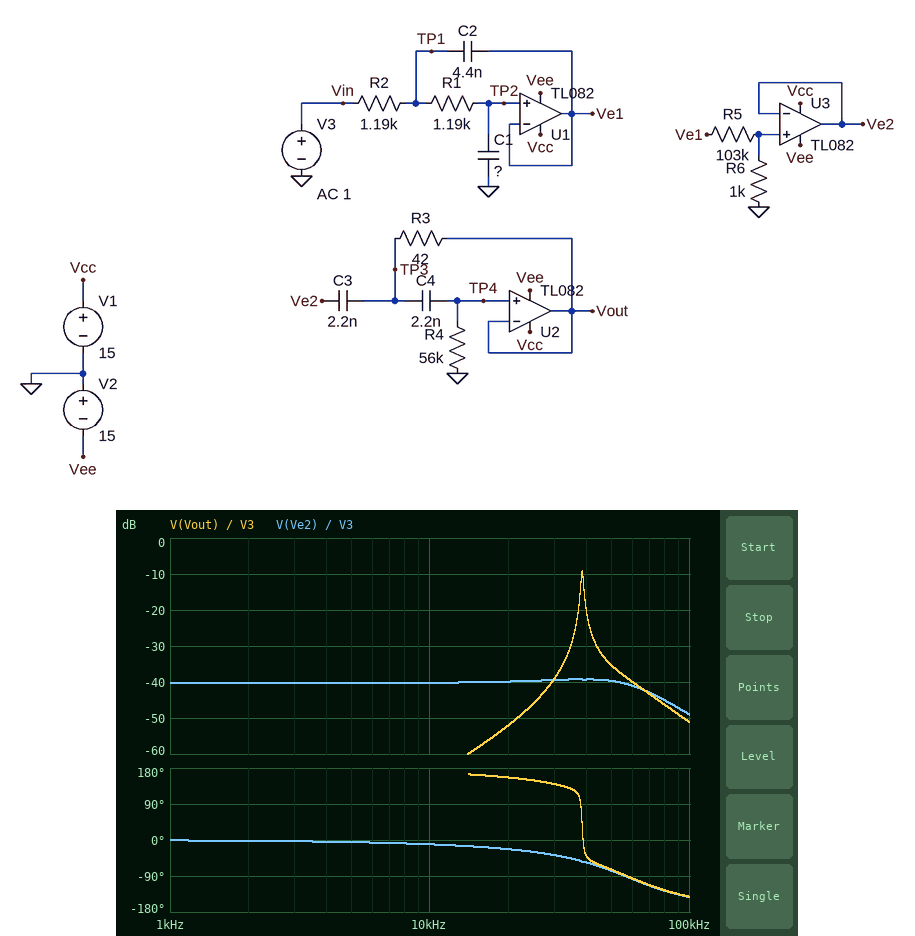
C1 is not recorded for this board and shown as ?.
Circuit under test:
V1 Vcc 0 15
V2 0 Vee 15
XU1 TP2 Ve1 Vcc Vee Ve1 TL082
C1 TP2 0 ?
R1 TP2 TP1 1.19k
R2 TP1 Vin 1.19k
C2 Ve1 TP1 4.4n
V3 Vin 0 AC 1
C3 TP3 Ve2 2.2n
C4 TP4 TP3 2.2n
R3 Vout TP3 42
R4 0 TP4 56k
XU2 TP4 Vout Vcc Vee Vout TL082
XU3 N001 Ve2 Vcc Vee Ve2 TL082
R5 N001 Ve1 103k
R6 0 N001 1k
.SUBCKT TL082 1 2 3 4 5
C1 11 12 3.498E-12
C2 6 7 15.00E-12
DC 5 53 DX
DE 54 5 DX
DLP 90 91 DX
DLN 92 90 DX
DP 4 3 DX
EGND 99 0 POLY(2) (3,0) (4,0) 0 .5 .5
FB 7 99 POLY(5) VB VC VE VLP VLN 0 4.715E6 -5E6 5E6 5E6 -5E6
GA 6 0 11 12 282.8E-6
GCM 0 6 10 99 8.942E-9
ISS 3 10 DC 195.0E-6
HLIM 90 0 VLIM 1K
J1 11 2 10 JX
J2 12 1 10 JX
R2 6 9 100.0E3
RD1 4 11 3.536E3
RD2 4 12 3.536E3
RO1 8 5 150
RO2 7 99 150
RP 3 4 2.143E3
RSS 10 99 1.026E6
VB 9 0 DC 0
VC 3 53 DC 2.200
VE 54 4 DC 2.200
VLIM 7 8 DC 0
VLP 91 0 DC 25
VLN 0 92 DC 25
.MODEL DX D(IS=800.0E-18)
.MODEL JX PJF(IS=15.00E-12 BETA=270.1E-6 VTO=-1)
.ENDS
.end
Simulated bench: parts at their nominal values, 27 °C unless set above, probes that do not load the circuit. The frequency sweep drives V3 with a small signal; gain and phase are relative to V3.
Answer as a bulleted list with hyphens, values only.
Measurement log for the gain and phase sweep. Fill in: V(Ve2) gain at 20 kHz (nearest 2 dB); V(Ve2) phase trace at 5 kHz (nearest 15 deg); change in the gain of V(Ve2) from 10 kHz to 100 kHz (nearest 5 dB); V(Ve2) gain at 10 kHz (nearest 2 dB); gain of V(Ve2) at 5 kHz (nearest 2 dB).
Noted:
- -40 dB
- 0 deg
- -10 dB
- -40 dB
- -40 dB
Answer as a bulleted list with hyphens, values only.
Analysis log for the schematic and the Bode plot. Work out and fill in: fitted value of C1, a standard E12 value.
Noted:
- 1.2 nF
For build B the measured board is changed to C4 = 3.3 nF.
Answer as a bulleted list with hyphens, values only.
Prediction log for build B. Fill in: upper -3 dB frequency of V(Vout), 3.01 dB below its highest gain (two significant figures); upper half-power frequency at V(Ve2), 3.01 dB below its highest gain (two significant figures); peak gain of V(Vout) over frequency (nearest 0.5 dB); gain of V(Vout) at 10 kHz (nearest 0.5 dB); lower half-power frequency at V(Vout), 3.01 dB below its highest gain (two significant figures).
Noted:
- 32 kHz
- 67 kHz
- -11.5 dB
- -62.5 dB
- 31 kHz
